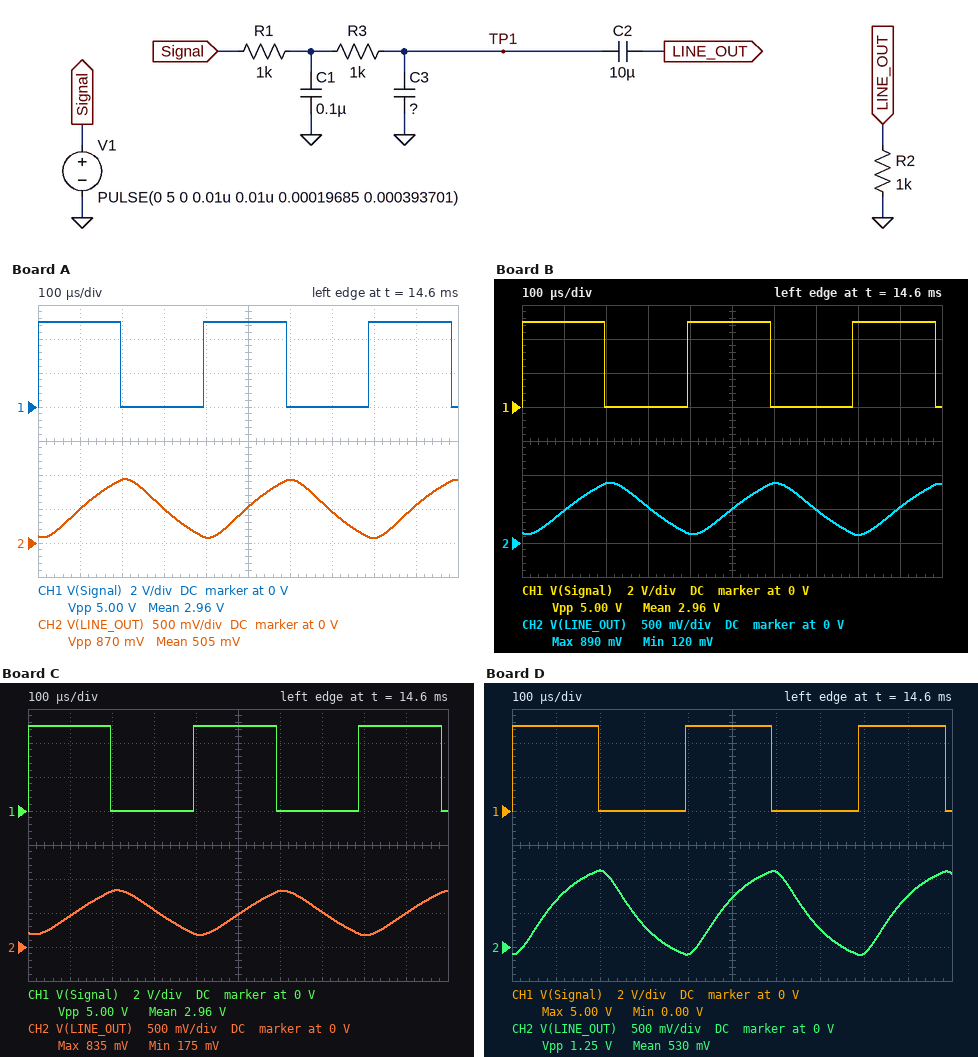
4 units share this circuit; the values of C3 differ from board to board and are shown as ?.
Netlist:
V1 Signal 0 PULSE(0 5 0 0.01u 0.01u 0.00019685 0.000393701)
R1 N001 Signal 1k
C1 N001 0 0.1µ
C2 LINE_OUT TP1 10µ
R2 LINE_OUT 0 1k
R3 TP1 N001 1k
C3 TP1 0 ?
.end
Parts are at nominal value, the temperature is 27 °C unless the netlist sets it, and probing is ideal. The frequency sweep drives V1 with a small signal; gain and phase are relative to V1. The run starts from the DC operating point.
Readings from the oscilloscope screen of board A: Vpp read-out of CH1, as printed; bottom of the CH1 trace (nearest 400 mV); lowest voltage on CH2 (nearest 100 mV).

5.00 V
0 V
100 mV
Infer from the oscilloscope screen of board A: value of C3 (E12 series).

150 nF
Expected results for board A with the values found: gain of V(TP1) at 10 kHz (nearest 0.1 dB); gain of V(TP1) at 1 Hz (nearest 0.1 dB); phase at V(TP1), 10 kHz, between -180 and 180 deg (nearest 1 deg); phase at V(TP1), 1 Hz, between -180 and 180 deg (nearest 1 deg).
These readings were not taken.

-36.2 dB
-0.1 dB
-151 deg
-7 deg
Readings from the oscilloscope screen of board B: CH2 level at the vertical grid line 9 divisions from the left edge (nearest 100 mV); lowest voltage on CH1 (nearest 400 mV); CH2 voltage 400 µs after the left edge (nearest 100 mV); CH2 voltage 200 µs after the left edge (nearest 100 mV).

500 mV
0 V
100 mV
900 mV
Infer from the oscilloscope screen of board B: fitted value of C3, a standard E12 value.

180 nF
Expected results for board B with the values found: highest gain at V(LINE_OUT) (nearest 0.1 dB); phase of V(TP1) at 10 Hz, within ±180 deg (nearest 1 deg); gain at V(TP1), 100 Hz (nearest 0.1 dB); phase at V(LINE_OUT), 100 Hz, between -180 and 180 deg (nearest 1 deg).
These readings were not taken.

-9.7 dB
-31 deg
-9.6 dB
-4 deg
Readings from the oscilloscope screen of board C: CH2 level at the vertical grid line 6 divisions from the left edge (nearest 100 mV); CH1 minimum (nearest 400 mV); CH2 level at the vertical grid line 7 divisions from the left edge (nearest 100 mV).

800 mV
0 V
500 mV
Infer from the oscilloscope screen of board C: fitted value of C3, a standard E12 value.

220 nF
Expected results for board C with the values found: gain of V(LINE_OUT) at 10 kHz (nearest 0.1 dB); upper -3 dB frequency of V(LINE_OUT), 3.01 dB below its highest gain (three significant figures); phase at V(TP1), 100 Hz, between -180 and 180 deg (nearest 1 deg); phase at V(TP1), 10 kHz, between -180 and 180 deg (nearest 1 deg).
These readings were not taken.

-39.4 dB
901 Hz
-14 deg
-154 deg
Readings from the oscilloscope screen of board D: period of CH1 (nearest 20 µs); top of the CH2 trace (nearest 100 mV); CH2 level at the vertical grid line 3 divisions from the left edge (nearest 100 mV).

400 µs
1.1 V
300 mV
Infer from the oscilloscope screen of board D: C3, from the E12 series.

68 nF
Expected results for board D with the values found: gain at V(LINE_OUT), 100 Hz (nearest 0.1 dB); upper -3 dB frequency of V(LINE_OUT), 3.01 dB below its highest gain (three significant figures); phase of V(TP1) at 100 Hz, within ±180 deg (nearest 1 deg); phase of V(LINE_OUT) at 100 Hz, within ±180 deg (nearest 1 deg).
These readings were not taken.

-9.6 dB
1.73 kHz
-10 deg
-1 deg
